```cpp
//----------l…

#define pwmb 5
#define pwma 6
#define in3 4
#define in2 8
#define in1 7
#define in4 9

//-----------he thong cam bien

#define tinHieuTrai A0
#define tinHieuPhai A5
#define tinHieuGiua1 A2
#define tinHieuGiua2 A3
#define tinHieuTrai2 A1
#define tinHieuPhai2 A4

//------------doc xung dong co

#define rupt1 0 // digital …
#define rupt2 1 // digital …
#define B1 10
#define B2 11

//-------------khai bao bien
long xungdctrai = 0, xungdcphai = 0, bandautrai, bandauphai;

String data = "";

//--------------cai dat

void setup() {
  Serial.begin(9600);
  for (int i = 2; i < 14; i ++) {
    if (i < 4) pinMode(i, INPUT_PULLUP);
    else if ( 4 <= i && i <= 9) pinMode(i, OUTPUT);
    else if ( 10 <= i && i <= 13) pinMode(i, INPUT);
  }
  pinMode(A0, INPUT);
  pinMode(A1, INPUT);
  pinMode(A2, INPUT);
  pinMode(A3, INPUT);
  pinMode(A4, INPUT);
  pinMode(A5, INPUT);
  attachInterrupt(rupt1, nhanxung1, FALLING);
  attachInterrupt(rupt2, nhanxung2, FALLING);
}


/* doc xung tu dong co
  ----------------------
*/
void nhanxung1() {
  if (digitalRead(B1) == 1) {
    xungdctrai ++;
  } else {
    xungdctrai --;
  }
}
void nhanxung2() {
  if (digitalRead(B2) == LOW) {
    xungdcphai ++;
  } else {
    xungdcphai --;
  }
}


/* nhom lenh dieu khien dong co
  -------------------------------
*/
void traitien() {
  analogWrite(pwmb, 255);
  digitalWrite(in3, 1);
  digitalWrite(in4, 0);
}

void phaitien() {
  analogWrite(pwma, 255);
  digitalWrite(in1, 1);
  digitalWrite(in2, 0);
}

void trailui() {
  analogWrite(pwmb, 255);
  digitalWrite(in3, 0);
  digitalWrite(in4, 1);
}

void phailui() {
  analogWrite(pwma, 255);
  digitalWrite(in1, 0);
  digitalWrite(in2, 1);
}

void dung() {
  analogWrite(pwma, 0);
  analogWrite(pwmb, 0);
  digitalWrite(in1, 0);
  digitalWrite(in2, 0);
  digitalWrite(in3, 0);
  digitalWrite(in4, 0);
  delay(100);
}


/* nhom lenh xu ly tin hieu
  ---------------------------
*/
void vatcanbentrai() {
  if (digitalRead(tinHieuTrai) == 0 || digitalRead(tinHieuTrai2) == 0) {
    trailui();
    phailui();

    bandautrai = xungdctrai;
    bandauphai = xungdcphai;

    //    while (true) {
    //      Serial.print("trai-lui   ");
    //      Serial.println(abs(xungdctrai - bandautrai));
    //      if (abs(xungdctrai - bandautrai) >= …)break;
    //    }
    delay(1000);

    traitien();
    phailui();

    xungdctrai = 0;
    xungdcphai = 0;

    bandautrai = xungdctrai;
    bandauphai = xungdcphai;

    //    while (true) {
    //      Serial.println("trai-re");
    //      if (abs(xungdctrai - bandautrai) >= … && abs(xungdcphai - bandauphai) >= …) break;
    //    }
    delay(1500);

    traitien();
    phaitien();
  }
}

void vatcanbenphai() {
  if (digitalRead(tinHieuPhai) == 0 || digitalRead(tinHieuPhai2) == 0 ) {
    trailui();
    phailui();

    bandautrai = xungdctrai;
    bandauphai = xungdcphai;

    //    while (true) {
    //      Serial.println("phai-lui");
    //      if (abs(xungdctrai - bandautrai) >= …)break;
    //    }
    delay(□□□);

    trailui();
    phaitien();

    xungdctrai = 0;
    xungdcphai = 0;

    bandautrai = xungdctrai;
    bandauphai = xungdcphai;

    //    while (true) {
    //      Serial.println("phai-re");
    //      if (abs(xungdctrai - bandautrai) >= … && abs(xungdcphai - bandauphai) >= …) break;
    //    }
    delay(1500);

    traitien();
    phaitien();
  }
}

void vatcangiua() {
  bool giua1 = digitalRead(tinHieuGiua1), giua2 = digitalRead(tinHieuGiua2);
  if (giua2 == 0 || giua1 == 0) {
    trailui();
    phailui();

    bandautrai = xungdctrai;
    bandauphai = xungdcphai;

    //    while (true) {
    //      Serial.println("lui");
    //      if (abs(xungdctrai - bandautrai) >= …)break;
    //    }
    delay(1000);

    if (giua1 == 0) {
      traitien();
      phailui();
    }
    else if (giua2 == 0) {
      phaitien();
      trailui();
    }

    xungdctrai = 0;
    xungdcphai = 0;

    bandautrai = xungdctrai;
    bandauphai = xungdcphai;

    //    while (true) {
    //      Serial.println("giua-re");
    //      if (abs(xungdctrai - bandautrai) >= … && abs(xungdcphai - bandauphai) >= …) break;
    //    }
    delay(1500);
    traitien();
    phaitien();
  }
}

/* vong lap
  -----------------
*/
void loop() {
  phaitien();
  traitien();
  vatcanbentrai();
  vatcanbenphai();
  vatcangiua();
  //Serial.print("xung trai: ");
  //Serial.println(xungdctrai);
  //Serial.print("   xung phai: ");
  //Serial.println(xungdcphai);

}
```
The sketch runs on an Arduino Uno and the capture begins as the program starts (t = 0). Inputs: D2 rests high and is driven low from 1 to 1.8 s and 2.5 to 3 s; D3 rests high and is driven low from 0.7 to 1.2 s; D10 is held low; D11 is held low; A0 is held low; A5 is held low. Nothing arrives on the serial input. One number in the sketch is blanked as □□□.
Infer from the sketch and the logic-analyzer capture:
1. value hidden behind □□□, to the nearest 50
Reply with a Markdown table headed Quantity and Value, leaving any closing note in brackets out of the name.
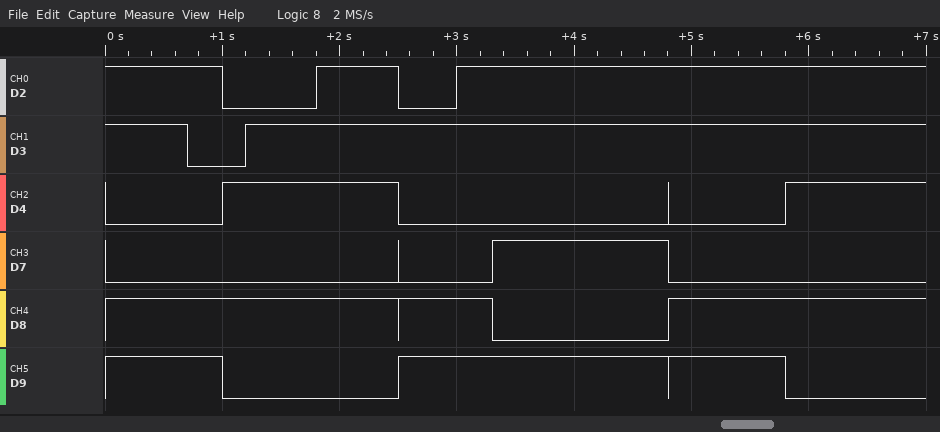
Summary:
| Quantity | Value |
|---|---|
| value hidden behind □□□, to the nearest 50 | 800 |
